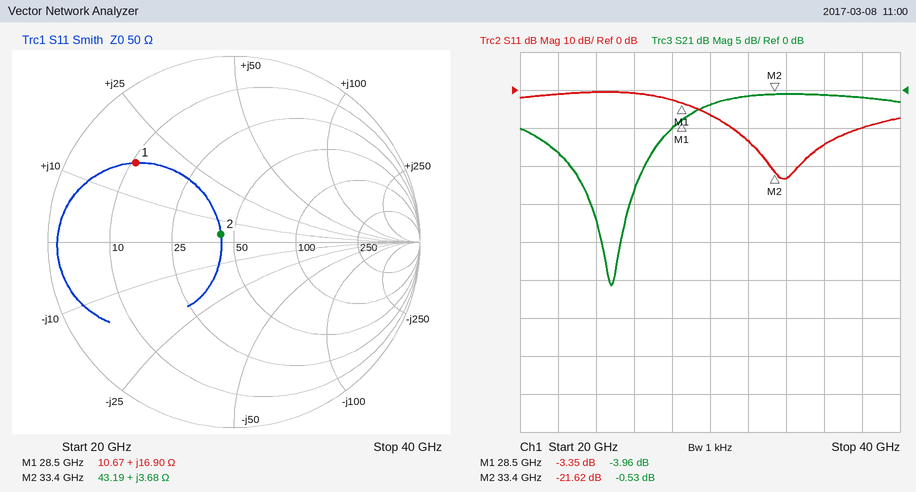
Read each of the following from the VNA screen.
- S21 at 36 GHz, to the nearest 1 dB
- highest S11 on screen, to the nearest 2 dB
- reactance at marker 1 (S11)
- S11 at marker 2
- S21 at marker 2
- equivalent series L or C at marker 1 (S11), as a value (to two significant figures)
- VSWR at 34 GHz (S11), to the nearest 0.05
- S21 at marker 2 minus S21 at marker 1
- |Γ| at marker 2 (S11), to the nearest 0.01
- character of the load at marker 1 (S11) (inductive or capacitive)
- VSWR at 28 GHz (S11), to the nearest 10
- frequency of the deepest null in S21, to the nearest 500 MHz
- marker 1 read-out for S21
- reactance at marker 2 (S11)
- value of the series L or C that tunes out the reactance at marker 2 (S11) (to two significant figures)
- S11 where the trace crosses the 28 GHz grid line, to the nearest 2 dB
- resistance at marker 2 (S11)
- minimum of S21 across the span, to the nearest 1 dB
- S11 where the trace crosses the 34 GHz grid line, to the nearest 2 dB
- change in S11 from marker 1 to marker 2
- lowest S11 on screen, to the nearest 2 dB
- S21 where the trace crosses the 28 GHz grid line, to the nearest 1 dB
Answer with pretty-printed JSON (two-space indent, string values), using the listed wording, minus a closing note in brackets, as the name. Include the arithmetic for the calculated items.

{
  "S21 at 36 GHz, to the nearest 1 dB": "-1 dB",
  "highest S11 on screen, to the nearest 2 dB": "0 dB",
  "reactance at marker 1": "+16.90 Ω",
  "S11 at marker 2": "-21.62 dB",
  "S21 at marker 2": "-0.53 dB",
  "equivalent series L or C at marker 1 (S11), as a value": "L = 16.9 Ω/(2π × 28.5 GHz) ≈ 94 pH",
  "VSWR at 34 GHz (S11), to the nearest 0.05": "|Γ| = 10^(-24/20) = 0.0631; VSWR = (1 + 0.0631)/(1 − 0.0631) ≈ 1.13, so 1.15 to the nearest 0.05",
  "S21 at marker 2 minus S21 at marker 1": "-0.53 − (-3.96) = 3.43 dB",
  "|Γ| at marker 2 (S11), to the nearest 0.01": "0.08",
  "character of the load at marker 1 (S11)": "inductive",
  "VSWR at 28 GHz (S11), to the nearest 10": "|Γ| = 10^(-2/20) = 0.7943; VSWR = (1 + 0.7943)/(1 − 0.7943) ≈ 8.72, so 10 to the nearest 10",
  "frequency of the deepest null in S21, to the nearest 500 MHz": "25.0 GHz",
  "marker 1 read-out for S21": "-3.96 dB",
  "reactance at marker 2": "+3.68 Ω",
  "value of the series L or C that tunes out the reactance at marker 2 (S11)": "C = 1/(2π × 33.4 GHz × 3.68 Ω) ≈ 1.3 pF",
  "S11 where the trace crosses the 28 GHz grid line, to the nearest 2 dB": "-2 dB",
  "resistance at marker 2": "43.19 Ω",
  "minimum of S21 across the span, to the nearest 1 dB": "-26 dB",
  "S11 where the trace crosses the 34 GHz grid line, to the nearest 2 dB": "-24 dB",
  "change in S11 from marker 1 to marker 2": "-21.62 − (-3.35) = -18.27 dB",
  "lowest S11 on screen, to the nearest 2 dB": "-24 dB",
  "S21 where the trace crosses the 28 GHz grid line, to the nearest 1 dB": "-5 dB"
}
